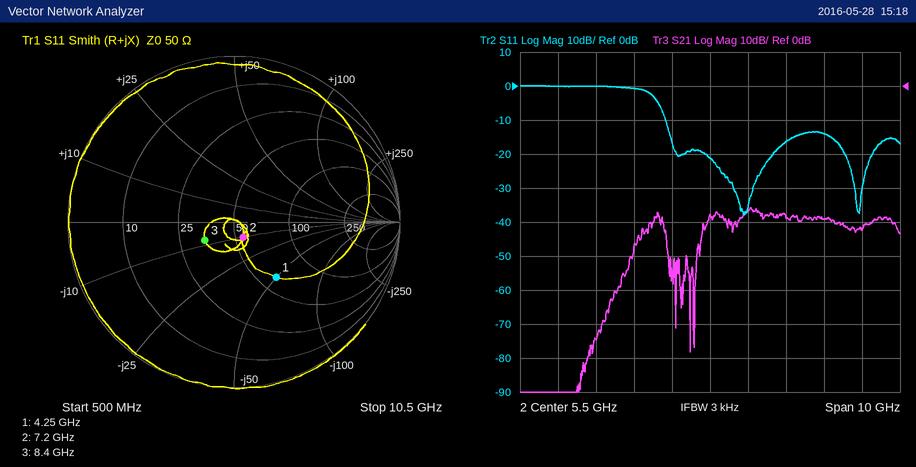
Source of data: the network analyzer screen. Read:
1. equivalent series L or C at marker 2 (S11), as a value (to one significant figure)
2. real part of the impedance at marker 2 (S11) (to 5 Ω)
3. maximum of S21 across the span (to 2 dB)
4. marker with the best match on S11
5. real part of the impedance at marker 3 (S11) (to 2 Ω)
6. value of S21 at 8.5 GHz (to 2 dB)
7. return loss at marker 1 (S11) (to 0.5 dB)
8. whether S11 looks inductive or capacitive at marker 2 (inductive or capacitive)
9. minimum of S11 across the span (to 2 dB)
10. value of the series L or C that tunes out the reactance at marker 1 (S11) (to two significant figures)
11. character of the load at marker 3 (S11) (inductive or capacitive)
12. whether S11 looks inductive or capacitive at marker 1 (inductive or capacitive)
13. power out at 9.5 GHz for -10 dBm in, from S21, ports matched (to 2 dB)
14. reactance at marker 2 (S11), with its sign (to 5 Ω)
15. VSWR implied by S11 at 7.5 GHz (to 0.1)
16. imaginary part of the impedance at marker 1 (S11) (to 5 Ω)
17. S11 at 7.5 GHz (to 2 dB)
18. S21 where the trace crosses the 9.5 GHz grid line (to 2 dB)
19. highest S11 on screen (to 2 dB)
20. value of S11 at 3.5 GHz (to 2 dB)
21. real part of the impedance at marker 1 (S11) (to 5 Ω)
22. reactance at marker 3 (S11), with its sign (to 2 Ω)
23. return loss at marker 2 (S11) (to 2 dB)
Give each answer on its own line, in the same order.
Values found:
2 pF
55 Ω
-36 dB
marker 2
34 Ω
-40 dB
7.5 dB
capacitive
-38 dB
1.9 nH
capacitive
capacitive
-52 dBm
-10 Ω
1.4
-50 Ω
-16 dB
-42 dB
0 dB
0 dB
60 Ω
-8 Ω
20 dB
